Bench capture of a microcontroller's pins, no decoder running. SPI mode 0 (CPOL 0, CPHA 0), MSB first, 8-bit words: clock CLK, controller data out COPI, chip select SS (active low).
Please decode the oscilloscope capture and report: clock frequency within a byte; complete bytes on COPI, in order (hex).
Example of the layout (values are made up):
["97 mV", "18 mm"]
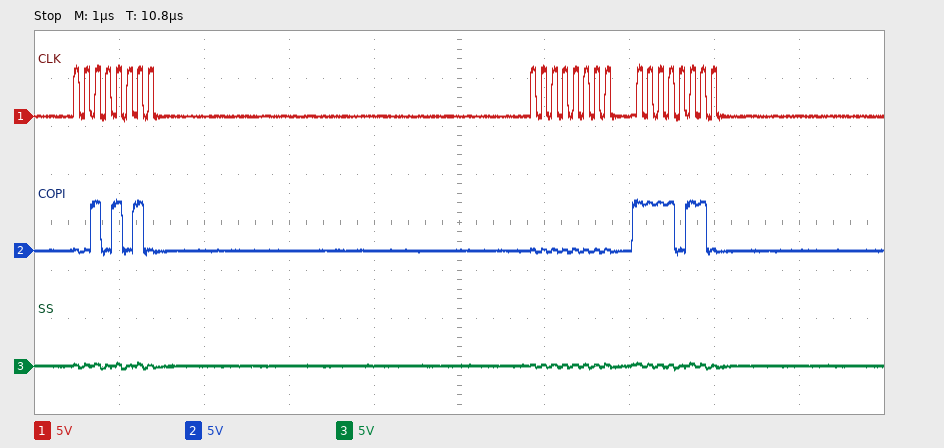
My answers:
["8 MHz", "2A 00 F6"]
